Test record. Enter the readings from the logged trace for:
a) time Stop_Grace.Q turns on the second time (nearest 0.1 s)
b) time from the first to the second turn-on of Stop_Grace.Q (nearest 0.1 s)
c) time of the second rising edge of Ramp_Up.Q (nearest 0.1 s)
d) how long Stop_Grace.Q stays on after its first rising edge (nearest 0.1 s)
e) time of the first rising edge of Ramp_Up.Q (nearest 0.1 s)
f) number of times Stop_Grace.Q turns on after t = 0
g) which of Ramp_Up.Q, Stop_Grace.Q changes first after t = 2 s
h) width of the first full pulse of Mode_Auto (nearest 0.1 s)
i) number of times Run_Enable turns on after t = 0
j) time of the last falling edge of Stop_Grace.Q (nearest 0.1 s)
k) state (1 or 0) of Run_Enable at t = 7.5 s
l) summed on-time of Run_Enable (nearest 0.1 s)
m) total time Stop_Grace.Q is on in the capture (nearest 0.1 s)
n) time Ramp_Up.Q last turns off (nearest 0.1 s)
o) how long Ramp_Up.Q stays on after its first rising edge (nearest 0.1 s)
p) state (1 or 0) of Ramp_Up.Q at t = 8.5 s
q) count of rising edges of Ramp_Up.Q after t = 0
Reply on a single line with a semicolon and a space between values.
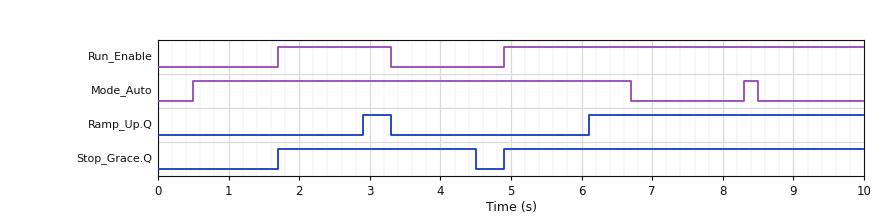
4.9 s; 3.2 s; 6.1 s; 2.8 s; 2.9 s; 2; Ramp_Up.Q; 6.2 s; 2; 4.5 s; 1; 6.7 s; 7.9 s; 3.3 s; 0.4 s; 1; 2
